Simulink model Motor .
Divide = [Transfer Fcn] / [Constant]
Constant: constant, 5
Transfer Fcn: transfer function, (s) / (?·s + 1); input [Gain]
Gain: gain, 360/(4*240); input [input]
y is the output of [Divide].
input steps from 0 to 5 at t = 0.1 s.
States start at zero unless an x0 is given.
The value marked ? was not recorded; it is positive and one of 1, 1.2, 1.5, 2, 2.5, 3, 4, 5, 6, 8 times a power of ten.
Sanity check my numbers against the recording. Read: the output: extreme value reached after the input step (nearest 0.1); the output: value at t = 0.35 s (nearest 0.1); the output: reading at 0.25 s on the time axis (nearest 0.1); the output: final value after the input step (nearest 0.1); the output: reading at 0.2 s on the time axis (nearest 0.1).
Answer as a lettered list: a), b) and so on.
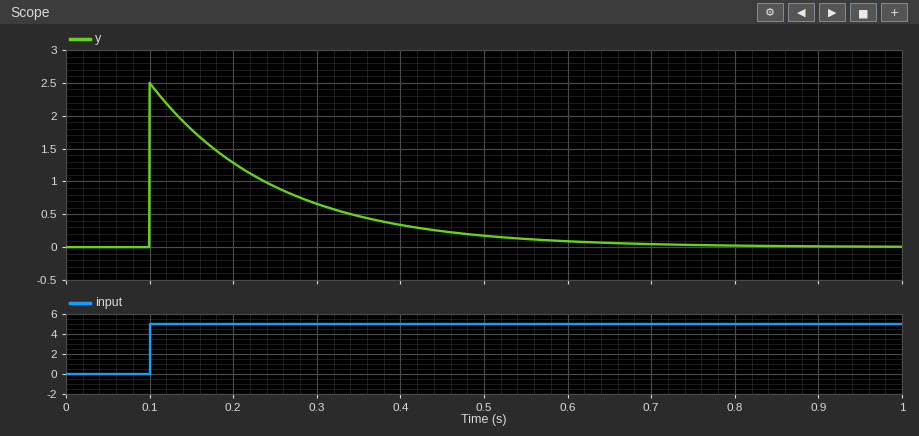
a) 2.5
b) 0.5
c) 0.9
d) 0.0
e) 1.3
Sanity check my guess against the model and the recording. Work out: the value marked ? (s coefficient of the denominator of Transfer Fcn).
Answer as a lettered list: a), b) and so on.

a) 0.15
